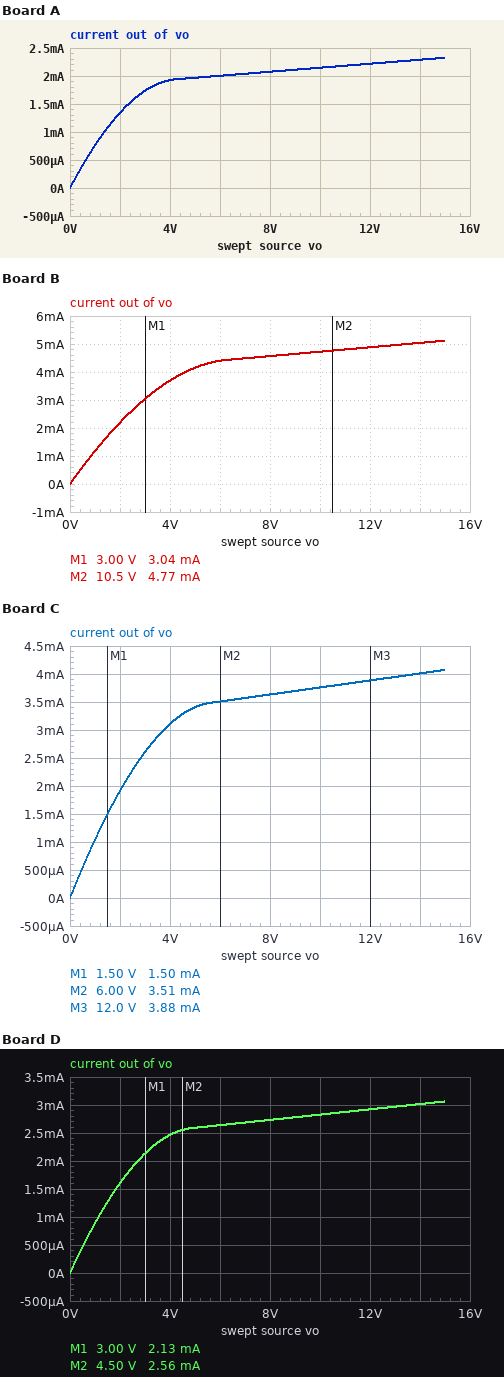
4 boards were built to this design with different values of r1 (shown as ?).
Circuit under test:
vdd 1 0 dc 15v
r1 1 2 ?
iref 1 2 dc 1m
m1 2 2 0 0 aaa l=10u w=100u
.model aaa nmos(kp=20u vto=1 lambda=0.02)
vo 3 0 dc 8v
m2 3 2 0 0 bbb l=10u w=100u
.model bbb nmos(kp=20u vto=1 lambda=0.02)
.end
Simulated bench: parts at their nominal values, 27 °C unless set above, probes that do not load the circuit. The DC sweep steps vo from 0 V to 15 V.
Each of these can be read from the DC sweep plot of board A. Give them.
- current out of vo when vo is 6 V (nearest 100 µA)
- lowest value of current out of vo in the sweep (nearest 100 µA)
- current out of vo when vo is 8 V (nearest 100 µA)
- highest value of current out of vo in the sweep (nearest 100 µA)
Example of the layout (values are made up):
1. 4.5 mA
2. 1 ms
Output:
1. 2.0 mA
2. 0 A
3. 2.1 mA
4. 2.3 mA
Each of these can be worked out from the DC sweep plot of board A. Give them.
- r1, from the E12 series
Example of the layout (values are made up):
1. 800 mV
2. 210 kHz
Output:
1. 10 kΩ
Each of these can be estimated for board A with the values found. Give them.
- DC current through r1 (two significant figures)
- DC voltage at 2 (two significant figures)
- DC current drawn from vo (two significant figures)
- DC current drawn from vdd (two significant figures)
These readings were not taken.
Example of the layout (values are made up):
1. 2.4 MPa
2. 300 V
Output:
1. 980 µA
2. 5.2 V
3. 2.1 mA
4. 2.0 mA
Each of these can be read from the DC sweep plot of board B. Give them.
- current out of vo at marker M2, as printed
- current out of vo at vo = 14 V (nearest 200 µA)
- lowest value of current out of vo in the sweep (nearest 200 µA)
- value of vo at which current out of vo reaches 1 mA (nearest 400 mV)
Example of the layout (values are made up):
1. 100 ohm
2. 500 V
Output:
1. 4.77 mA
2. 5.0 mA
3. 0 A
4. 800 mV
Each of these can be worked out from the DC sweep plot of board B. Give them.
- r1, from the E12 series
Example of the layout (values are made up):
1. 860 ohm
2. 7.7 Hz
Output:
1. 2.2 kΩ
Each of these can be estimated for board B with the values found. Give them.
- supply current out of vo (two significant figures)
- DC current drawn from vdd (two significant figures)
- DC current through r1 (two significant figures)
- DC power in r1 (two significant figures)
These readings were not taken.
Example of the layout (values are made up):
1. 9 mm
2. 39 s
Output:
1. 4.6 mA
2. 4.5 mA
3. 3.5 mA
4. 27 mW
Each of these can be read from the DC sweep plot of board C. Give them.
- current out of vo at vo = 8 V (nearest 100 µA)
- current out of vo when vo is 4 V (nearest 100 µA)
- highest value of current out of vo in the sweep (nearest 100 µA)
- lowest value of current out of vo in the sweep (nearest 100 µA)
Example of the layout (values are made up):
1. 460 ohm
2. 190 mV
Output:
1. 3.6 mA
2. 3.1 mA
3. 4.1 mA
4. 0 A
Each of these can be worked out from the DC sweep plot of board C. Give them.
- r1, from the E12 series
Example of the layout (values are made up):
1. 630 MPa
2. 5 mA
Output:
1. 3.3 kΩ
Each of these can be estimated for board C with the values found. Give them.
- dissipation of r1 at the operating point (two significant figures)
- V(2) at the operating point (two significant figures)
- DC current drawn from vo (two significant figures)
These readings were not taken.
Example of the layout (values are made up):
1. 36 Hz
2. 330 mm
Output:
1. 21 mW
2. 6.6 V
3. 3.6 mA
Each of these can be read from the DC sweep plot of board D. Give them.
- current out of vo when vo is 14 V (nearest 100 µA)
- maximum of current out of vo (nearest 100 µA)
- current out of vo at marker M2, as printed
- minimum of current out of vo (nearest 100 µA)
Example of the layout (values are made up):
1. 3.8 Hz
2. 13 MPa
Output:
1. 3.0 mA
2. 3.1 mA
3. 2.56 mA
4. 0 A
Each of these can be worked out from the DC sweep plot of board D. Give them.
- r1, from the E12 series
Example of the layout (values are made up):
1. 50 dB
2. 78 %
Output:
1. 5.6 kΩ
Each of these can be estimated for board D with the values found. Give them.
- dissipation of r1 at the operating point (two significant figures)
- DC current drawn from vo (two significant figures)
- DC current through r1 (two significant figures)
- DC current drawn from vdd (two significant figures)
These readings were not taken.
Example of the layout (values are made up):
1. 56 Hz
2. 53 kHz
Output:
1. 15 mW
2. 2.7 mA
3. 1.6 mA
4. 2.6 mA
